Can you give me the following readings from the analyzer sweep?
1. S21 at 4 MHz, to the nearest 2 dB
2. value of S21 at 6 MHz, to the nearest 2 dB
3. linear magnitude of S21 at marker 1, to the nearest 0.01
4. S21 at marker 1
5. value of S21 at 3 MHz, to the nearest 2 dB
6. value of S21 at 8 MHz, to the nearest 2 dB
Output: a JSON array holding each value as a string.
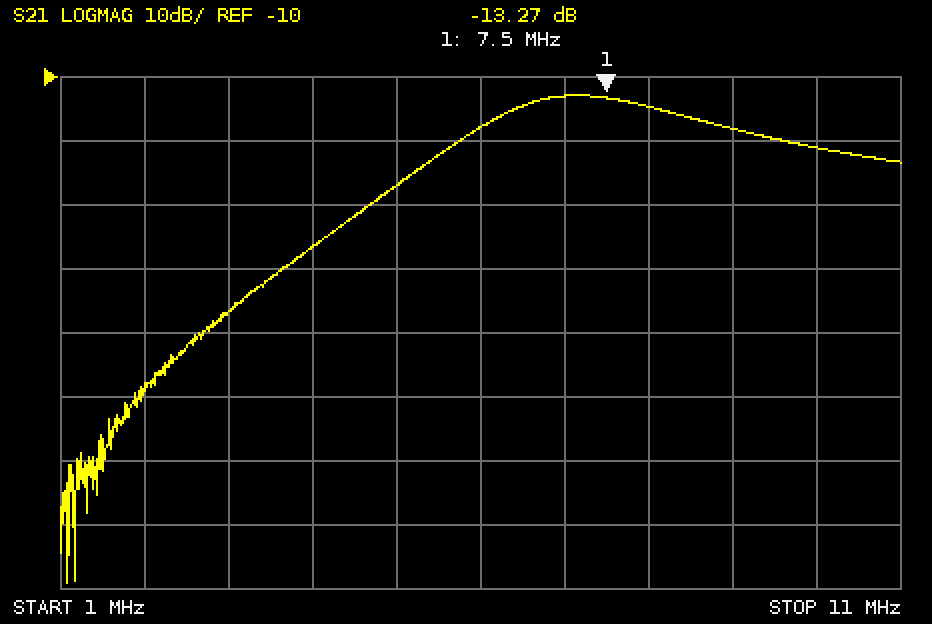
["-36 dB", "-18 dB", "0.22", "-13.27 dB", "-46 dB", "-14 dB"]
